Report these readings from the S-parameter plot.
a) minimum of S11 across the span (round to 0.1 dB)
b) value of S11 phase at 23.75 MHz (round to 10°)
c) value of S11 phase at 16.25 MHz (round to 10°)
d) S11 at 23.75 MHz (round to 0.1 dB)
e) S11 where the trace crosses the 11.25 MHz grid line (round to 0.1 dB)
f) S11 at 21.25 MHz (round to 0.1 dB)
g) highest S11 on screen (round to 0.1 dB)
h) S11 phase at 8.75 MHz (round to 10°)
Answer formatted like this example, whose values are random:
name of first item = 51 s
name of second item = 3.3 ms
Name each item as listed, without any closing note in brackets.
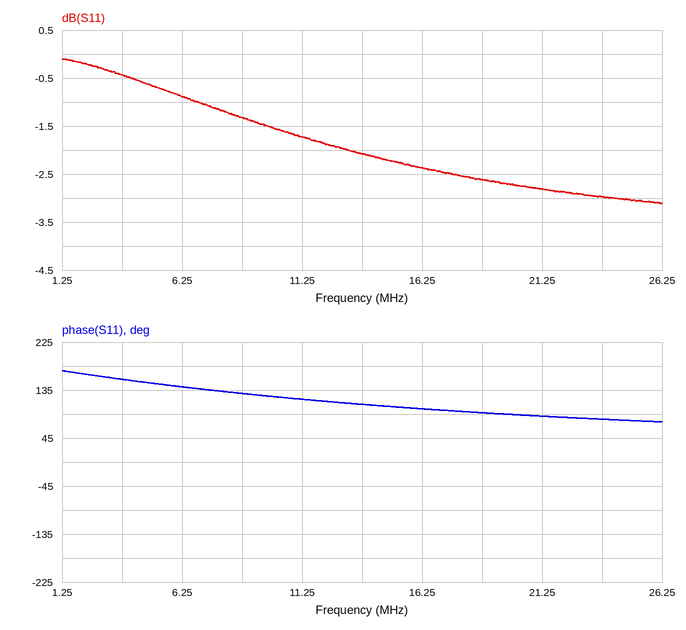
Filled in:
minimum of S11 across the span = -3.1 dB
value of S11 phase at 23.75 MHz = 80°
value of S11 phase at 16.25 MHz = 100°
S11 at 23.75 MHz = -3.0 dB
S11 where the trace crosses the 11.25 MHz grid line = -1.7 dB
S11 at 21.25 MHz = -2.8 dB
highest S11 on screen = -0.1 dB
S11 phase at 8.75 MHz = 130°
